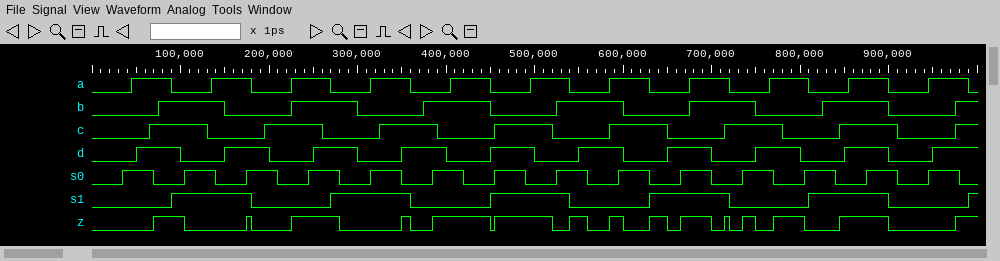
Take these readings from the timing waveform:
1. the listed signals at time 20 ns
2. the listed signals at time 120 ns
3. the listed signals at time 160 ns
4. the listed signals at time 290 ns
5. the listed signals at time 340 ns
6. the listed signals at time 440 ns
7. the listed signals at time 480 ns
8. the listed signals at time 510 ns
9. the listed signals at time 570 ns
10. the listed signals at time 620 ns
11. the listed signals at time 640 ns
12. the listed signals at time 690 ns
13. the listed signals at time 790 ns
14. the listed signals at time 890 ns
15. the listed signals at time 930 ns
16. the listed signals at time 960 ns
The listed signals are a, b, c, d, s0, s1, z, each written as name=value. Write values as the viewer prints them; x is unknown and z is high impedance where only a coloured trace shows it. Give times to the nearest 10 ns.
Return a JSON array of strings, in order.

["a=0, b=0, c=0, d=0, s0=0, s1=0, z=0", "a=0, b=1, c=1, d=0, s0=1, s1=1, z=0", "a=1, b=0, c=0, d=1, s0=0, s1=1, z=0", "a=0, b=1, c=0, d=1, s0=0, s1=1, z=0", "a=1, b=0, c=1, d=0, s0=1, s1=1, z=0", "a=1, b=1, c=0, d=0, s0=0, s1=0, z=1", "a=0, b=0, c=1, d=1, s0=1, s1=1, z=1", "a=1, b=0, c=1, d=0, s0=0, s1=1, z=1", "a=0, b=1, c=0, d=1, s0=0, s1=0, z=0", "a=1, b=0, c=1, d=0, s0=1, s1=0, z=0", "a=0, b=0, c=1, d=0, s0=0, s1=1, z=1", "a=1, b=1, c=0, d=1, s0=1, s1=1, z=1", "a=1, b=0, c=0, d=1, s0=0, s1=0, z=1", "a=1, b=1, c=1, d=1, s0=1, s1=1, z=1", "a=0, b=0, c=0, d=0, s0=0, s1=0, z=0", "a=1, b=0, c=0, d=1, s0=1, s1=0, z=0"]
